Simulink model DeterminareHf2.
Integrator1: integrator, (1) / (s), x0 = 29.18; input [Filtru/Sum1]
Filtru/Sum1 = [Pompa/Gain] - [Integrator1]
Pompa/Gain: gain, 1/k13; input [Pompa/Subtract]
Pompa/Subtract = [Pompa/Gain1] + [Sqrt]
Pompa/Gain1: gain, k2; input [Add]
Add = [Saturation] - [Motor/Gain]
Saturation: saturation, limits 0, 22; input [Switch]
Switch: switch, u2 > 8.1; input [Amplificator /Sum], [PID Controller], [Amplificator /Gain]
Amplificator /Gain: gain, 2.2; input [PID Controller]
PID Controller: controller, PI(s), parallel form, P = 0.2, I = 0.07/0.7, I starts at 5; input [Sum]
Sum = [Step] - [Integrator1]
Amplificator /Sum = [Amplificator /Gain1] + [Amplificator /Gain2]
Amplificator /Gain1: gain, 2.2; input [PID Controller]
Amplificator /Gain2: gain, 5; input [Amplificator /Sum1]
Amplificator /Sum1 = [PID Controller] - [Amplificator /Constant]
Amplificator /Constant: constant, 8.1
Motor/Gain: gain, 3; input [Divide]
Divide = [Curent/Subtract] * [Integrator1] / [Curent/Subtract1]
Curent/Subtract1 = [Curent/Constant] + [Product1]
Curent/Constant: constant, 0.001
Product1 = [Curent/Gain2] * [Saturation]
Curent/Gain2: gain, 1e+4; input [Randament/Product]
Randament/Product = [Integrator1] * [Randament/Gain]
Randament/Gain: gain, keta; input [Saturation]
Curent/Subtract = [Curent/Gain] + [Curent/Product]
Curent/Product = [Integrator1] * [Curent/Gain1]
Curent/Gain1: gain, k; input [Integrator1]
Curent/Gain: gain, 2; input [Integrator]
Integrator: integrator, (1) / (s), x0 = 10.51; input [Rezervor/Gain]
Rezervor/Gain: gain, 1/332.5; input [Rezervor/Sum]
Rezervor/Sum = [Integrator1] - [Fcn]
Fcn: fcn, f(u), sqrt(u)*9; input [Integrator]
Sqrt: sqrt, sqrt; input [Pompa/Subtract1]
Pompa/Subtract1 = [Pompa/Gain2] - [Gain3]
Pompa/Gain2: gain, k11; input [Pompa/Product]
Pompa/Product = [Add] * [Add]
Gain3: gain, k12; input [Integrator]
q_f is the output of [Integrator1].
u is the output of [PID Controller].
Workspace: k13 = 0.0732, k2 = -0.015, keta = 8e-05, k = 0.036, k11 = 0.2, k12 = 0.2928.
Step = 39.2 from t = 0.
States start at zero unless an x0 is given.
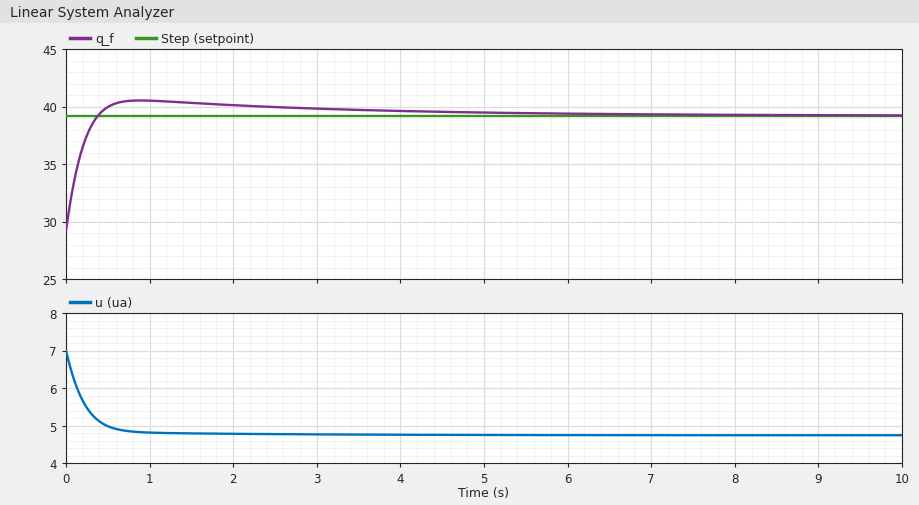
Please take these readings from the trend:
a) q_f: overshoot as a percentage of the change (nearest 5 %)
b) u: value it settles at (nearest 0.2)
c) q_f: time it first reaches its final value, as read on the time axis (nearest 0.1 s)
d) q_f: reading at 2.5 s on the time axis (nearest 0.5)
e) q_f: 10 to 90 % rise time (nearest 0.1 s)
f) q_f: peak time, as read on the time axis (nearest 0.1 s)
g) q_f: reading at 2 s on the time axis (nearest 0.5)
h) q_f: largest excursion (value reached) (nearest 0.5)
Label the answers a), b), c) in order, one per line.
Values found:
a) 15 %
b) 4.8
c) 0.4 s
d) 40.0
e) 0.3 s
f) 0.9 s
g) 40.0
h) 40.5
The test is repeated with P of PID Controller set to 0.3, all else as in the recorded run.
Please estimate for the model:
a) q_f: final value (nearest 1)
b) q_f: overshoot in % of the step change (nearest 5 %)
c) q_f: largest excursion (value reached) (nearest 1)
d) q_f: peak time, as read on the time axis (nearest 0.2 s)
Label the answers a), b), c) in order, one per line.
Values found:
a) 39
b) 10 %
c) 40
d) 0.8 s
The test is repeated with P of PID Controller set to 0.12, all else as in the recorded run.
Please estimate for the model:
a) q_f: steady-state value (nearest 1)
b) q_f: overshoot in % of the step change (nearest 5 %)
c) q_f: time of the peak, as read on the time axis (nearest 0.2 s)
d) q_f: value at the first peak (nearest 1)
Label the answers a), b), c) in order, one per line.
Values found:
a) 39
b) 20 %
c) 1.0 s
d) 41
